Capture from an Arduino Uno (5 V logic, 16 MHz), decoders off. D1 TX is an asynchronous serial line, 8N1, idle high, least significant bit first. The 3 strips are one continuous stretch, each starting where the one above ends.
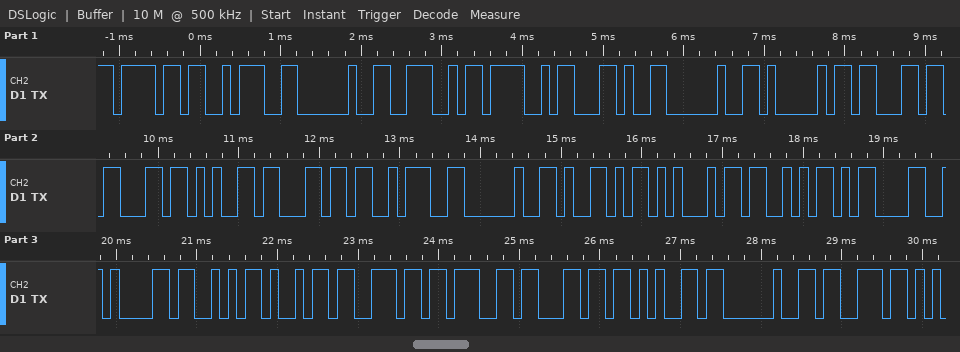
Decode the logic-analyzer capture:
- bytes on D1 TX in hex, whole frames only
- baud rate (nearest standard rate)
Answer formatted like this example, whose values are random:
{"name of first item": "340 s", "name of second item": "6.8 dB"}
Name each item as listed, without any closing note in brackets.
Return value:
{"bytes on D1 TX in hex, whole frames only": "6F 3A 20 4E 4F 2C 20 41 63 63 65 6C 3A 20 59 45 53 0D 0A 53 69 6E 67 6C 65 20 73", "baud rate": "9600 baud"}
